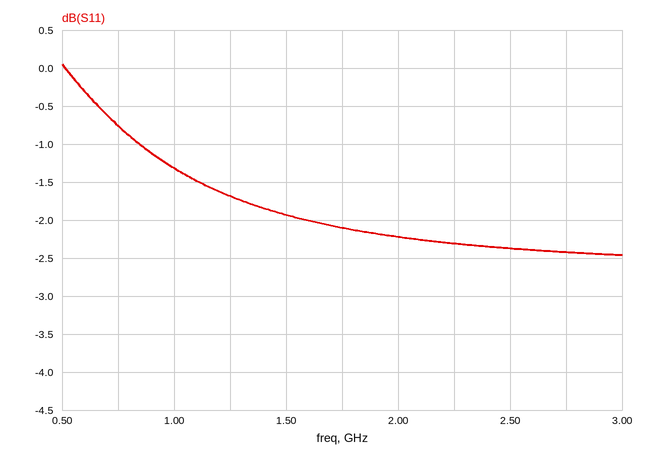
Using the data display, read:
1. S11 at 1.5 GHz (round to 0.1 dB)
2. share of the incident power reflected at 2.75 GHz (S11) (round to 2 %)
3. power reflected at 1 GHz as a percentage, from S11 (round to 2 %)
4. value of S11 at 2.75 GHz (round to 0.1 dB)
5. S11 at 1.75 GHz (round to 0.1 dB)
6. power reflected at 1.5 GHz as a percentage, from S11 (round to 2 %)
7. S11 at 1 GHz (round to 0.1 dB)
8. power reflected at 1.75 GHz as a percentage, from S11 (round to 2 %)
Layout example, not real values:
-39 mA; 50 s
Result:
-1.9 dB; 58 %; 74 %; -2.4 dB; -2.1 dB; 64 %; -1.3 dB; 62 %
